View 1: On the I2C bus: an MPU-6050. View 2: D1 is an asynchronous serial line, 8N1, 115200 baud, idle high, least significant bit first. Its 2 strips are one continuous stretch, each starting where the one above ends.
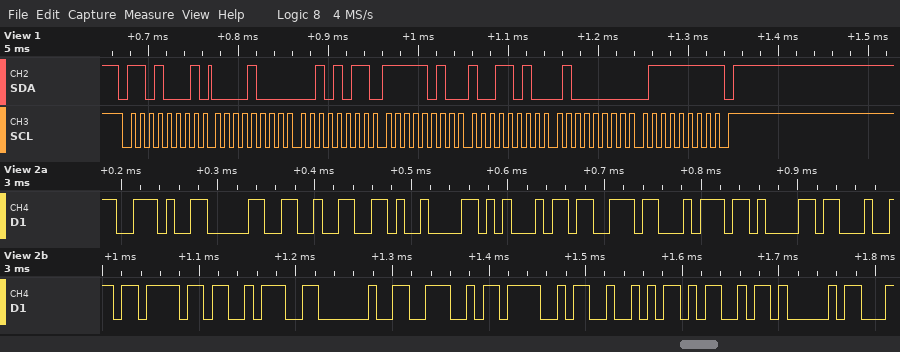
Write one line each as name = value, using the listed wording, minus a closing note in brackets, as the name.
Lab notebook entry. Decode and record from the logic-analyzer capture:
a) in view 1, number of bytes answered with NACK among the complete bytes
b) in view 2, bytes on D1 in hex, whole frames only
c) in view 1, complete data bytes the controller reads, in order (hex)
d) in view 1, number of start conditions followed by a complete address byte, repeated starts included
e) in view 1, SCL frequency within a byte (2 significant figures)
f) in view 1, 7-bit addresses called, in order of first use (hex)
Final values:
in view 1, number of bytes answered with NACK among the complete bytes = 1
in view 2, bytes on D1 in hex, whole frames only = 2E 30 32 09 45 73 74 61 64 6F 3A 20 4E 4F 52 4D 41
in view 1, complete data bytes the controller reads, in order = 08 2B FA 9A 40 7F
in view 1, number of start conditions followed by a complete address byte, repeated starts included = 1
in view 1, SCL frequency within a byte = 100 kHz
in view 1, 7-bit addresses called, in order of first use = 0x68
